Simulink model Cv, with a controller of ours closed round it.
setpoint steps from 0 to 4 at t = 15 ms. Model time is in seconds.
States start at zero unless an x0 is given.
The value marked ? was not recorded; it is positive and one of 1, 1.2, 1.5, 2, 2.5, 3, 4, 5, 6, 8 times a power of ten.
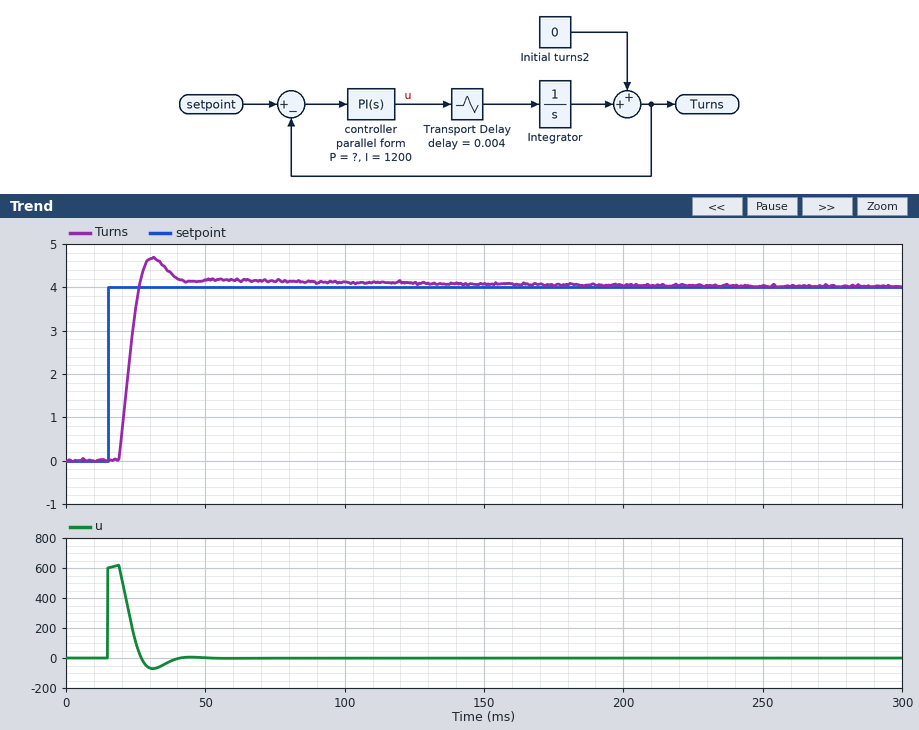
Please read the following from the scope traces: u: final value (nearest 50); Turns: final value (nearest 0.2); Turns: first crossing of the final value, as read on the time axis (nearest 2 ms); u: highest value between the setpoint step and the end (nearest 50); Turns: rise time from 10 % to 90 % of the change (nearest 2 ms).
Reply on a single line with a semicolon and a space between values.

0; 4.0; 26 ms; 600; 6 ms
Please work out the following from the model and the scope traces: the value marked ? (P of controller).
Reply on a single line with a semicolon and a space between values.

150
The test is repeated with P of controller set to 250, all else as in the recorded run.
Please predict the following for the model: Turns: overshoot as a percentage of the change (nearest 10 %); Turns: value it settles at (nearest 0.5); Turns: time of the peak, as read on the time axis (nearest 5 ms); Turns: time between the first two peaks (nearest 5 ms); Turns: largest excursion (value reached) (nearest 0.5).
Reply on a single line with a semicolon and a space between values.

50 %; 4.0; 25 ms; 20 ms; 6.0
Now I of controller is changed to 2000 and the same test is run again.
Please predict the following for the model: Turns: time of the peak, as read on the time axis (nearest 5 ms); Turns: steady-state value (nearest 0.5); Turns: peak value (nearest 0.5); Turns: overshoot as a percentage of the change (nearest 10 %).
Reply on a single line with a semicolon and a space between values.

30 ms; 4.0; 5.0; 20 %
